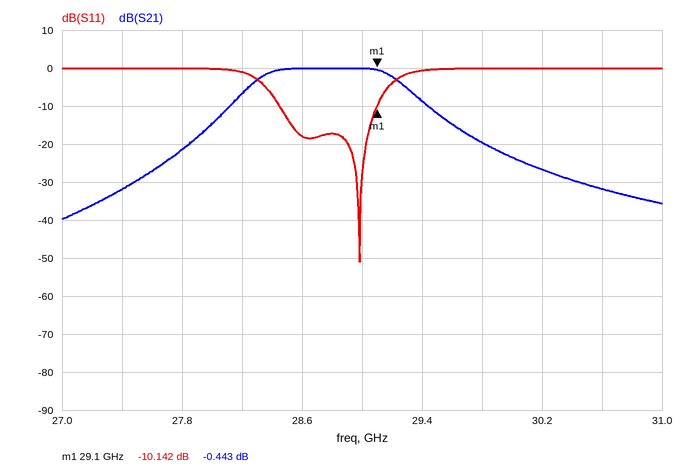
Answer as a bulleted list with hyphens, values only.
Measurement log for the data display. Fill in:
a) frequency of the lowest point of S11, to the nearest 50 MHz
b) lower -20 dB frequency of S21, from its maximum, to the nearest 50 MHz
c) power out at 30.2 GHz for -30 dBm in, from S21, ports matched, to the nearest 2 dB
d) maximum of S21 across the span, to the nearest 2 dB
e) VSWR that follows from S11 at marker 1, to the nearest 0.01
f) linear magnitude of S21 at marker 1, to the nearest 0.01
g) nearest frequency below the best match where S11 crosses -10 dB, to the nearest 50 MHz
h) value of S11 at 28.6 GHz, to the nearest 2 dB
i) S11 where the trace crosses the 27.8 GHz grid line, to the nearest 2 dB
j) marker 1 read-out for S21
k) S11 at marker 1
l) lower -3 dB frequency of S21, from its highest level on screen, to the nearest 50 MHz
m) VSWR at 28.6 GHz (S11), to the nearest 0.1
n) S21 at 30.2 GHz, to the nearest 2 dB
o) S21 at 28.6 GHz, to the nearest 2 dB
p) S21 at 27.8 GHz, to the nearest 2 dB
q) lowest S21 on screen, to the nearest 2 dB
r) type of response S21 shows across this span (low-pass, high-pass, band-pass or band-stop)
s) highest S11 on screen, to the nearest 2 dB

- 29.00 GHz
- 27.85 GHz
- -56 dBm
- 0 dB
- 1.90
- 0.95
- 28.45 GHz
- -18 dB
- 0 dB
- -0.443 dB
- -10.142 dB
- 28.30 GHz
- 1.3
- -26 dB
- 0 dB
- -22 dB
- -40 dB
- band-pass
- 0 dB
